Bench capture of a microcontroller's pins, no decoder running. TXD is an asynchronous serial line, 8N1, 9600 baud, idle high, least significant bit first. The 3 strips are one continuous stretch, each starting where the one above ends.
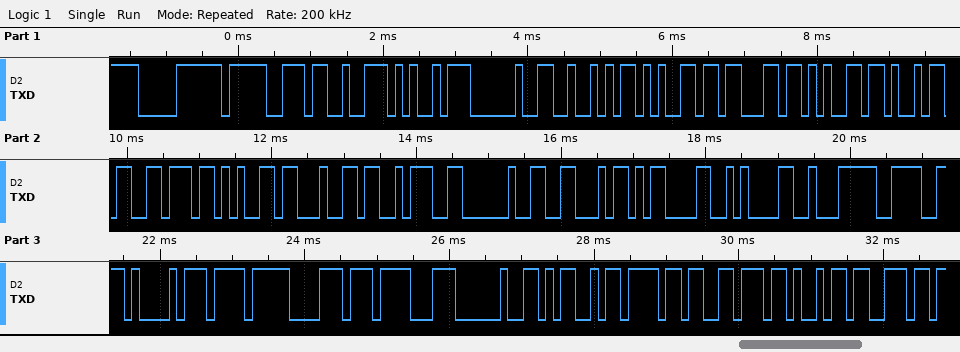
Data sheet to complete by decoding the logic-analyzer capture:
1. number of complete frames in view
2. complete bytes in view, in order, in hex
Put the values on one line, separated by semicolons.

30; F0 9F 93 A5 20 52 65 63 65 69 76 65 64 3A 20 46 0D 0A E2 9E A1 EF B8 8F 20 4D 6F 76 69 6E
